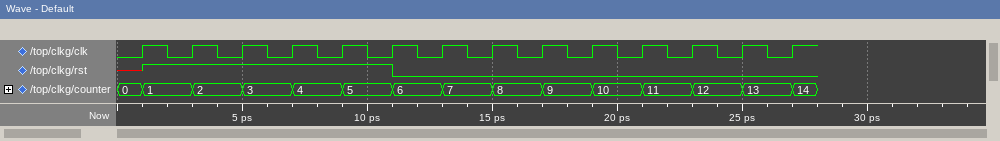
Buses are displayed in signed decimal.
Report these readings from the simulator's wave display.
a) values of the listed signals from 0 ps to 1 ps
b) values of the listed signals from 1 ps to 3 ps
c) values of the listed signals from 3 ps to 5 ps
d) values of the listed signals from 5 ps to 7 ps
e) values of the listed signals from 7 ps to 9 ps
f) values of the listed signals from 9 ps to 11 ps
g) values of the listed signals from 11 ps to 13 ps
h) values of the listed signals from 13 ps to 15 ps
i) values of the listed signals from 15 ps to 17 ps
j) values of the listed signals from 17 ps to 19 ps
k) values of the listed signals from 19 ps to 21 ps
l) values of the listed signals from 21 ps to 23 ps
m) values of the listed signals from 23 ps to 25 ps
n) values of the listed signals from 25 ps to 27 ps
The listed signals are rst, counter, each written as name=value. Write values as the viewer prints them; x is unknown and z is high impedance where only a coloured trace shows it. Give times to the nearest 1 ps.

rst=x, counter=0
rst=1, counter=1
rst=1, counter=2
rst=1, counter=3
rst=1, counter=4
rst=1, counter=5
rst=0, counter=6
rst=0, counter=7
rst=0, counter=8
rst=0, counter=9
rst=0, counter=10
rst=0, counter=11
rst=0, counter=12
rst=0, counter=13
